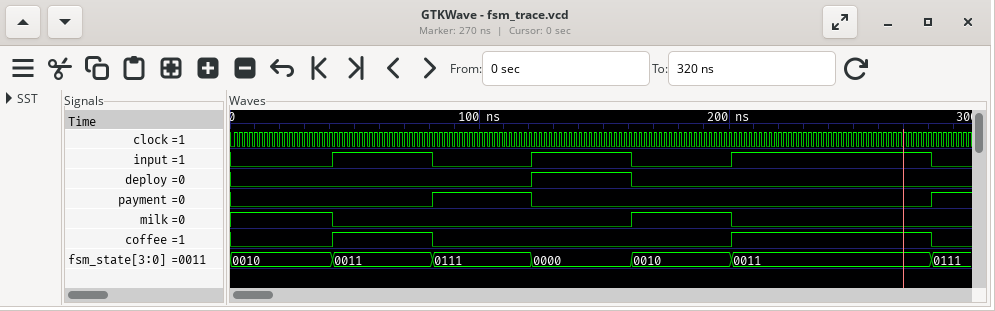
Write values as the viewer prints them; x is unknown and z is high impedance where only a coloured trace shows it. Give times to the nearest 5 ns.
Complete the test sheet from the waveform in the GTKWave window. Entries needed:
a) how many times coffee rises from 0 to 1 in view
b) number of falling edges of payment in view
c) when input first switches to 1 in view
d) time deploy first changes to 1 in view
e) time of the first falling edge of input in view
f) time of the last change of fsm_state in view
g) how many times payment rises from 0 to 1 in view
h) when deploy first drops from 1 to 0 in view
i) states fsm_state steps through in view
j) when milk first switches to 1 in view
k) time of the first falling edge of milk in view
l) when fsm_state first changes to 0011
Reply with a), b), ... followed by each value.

a) 2
b) 1
c) 40 ns
d) 120 ns
e) 80 ns
f) 280 ns
g) 2
h) 160 ns
i) 0010, 0011, 0111, 0000, 0010, 0011, 0111
j) 160 ns
k) 40 ns
l) 40 ns
